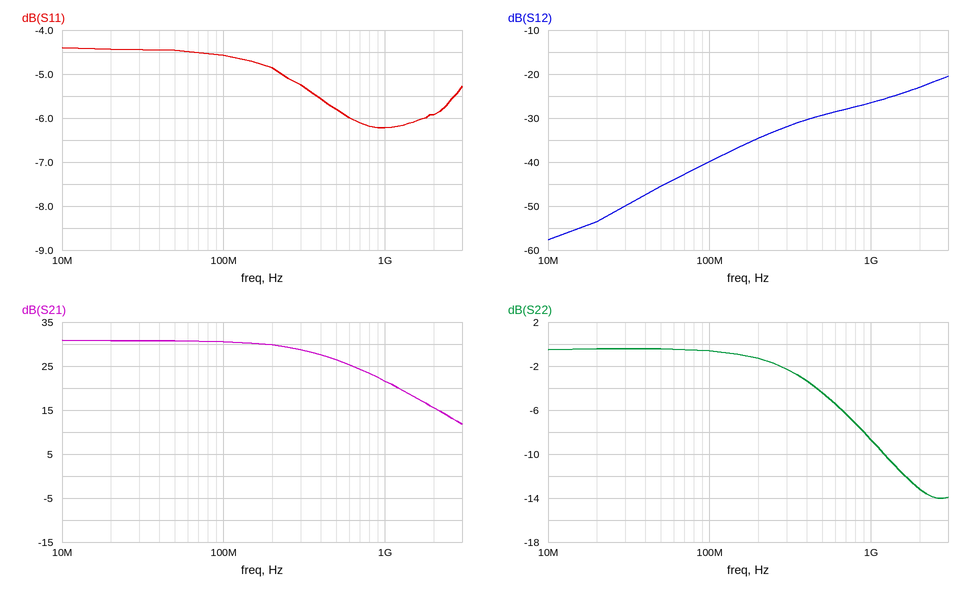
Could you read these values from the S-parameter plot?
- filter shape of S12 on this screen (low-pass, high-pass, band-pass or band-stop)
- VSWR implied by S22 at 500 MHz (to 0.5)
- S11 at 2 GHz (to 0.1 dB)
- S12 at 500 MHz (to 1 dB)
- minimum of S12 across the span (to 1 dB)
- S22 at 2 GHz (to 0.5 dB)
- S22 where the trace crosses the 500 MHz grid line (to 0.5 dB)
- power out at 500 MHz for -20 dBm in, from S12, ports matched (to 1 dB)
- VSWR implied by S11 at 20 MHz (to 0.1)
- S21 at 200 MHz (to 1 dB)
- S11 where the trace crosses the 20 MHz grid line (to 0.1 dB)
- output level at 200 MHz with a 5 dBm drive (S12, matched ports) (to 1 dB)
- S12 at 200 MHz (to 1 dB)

high-pass
4.0
-5.9 dB
-29 dB
-58 dB
-13.0 dB
-4.5 dB
-49 dBm
4.0
30 dB
-4.4 dB
-30 dBm
-35 dB
